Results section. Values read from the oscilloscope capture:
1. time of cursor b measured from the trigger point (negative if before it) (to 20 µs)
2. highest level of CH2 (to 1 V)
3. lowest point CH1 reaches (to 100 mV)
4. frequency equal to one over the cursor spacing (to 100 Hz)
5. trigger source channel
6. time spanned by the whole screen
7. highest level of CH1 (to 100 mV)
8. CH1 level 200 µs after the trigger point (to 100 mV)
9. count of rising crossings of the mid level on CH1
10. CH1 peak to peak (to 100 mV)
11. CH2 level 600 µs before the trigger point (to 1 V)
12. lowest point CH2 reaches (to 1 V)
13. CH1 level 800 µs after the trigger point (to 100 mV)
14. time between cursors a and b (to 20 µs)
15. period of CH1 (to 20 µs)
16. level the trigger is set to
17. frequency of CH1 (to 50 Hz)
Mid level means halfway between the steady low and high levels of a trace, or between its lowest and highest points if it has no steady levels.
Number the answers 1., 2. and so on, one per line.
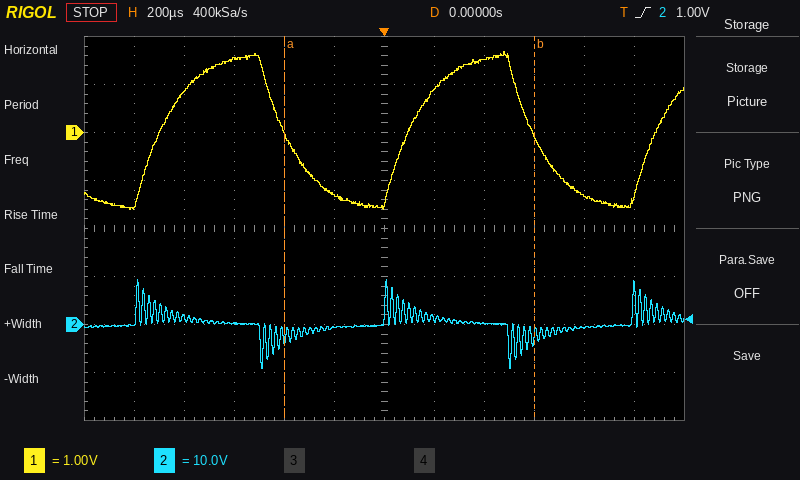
1. +600 µs
2. 9 V
3. -1.6 V
4. 1.0 kHz
5. CH2
6. 2.4 ms
7. 1.7 V
8. 900 mV
9. 3
10. 3.3 V
11. 0 V
12. -9 V
13. -1.3 V
14. 1.00 ms
15. 1.00 ms
16. 1.00 V
17. 1.00 kHz
